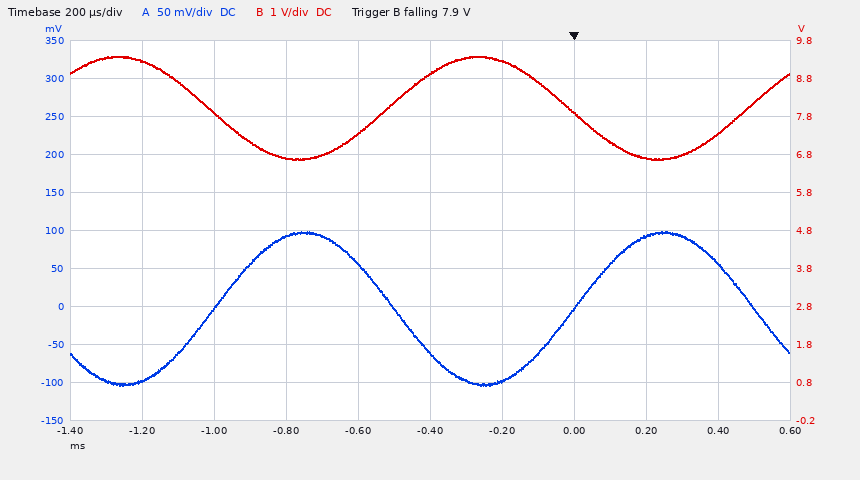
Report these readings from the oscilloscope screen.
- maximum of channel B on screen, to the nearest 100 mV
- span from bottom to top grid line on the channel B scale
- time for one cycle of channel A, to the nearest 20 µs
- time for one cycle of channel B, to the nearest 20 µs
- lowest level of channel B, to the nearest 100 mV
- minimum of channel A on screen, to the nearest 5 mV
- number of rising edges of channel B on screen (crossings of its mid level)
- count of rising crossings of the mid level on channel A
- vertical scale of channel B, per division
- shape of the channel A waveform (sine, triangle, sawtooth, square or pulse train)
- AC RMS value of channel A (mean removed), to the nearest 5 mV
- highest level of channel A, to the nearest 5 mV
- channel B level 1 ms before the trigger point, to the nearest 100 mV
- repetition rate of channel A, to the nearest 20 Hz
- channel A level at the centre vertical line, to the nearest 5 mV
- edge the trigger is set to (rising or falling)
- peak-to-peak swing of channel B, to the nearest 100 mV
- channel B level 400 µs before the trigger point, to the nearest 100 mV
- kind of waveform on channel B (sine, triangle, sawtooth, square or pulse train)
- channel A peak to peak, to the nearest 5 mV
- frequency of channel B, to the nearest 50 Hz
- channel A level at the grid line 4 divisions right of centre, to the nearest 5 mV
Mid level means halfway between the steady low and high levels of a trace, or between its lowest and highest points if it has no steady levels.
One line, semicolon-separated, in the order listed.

9.4 V; 10 V; 1.00 ms; 1.00 ms; 6.7 V; -105 mV; 2; 2; 1 V; sine; 70 mV; 100 mV; 7.9 V; 1.00 kHz; -60 mV; falling; 2.7 V; 8.9 V; sine; 205 mV; 1.00 kHz; 55 mV
